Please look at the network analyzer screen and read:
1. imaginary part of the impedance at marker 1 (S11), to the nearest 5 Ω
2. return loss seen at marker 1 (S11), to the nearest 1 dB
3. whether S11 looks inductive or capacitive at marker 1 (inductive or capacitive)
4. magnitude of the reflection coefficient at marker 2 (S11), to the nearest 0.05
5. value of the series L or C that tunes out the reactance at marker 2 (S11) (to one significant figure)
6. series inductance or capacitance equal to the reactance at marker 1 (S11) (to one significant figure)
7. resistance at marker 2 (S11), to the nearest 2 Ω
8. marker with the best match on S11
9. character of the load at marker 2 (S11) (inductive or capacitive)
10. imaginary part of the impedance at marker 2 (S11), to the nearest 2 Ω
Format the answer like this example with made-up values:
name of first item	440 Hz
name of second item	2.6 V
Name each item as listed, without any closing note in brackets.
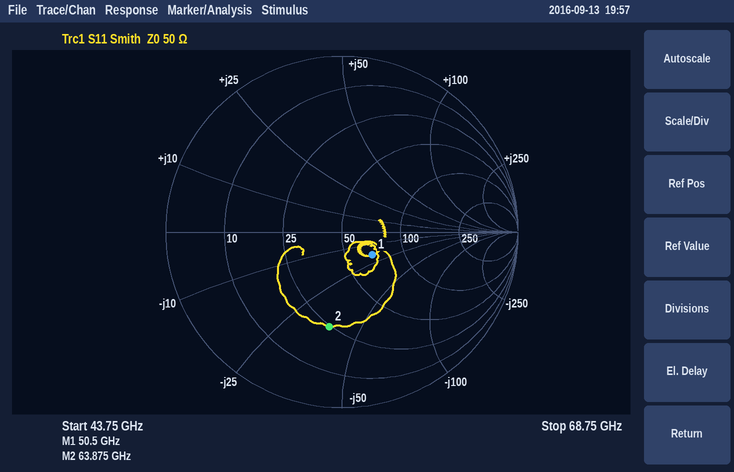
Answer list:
imaginary part of the impedance at marker 1 (S11), to the nearest 5 Ω	-20 Ω
return loss seen at marker 1 (S11), to the nearest 1 dB	13 dB
whether S11 looks inductive or capacitive at marker 1	capacitive
magnitude of the reflection coefficient at marker 2 (S11), to the nearest 0.05	0.55
value of the series L or C that tunes out the reactance at marker 2 (S11)	90 pH
series inductance or capacitance equal to the reactance at marker 1 (S11)	200 fF
resistance at marker 2 (S11), to the nearest 2 Ω	24 Ω
marker with the best match on S11	marker 1
character of the load at marker 2 (S11)	capacitive
imaginary part of the impedance at marker 2 (S11), to the nearest 2 Ω	-38 Ω
